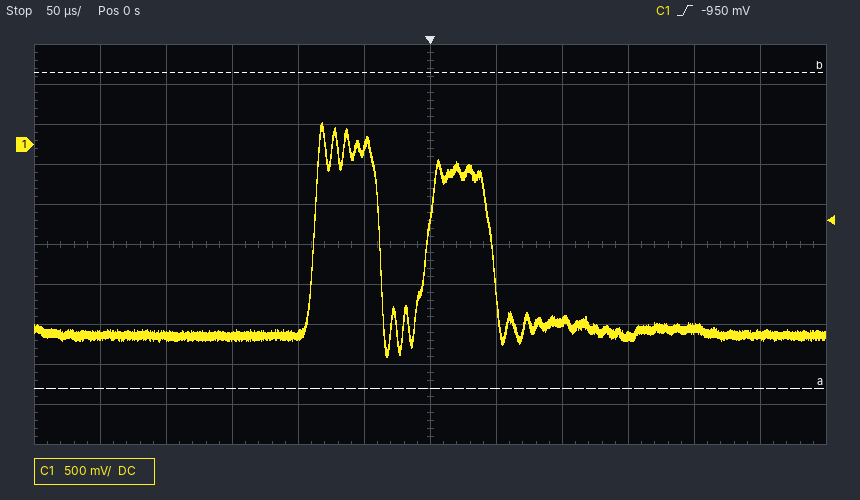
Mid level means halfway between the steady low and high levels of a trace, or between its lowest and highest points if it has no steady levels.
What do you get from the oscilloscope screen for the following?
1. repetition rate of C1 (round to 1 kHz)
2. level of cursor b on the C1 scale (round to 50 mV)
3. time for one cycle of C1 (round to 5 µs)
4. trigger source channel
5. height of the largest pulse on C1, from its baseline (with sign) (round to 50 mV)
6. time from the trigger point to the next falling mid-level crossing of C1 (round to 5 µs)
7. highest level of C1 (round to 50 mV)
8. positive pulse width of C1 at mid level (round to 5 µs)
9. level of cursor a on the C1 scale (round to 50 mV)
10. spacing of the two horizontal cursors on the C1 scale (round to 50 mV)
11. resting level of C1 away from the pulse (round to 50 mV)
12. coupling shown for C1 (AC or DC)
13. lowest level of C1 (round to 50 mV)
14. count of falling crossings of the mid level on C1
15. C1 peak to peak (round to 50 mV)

12 kHz
900 mV
85 µs
C1
+2.65 V
45 µs
250 mV
50 µs
-3.05 V
3.95 V
-2.40 V
DC
-2.65 V
2
2.90 V
